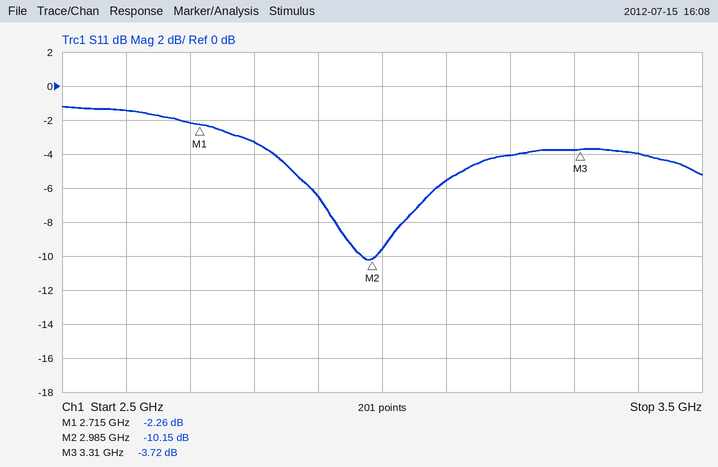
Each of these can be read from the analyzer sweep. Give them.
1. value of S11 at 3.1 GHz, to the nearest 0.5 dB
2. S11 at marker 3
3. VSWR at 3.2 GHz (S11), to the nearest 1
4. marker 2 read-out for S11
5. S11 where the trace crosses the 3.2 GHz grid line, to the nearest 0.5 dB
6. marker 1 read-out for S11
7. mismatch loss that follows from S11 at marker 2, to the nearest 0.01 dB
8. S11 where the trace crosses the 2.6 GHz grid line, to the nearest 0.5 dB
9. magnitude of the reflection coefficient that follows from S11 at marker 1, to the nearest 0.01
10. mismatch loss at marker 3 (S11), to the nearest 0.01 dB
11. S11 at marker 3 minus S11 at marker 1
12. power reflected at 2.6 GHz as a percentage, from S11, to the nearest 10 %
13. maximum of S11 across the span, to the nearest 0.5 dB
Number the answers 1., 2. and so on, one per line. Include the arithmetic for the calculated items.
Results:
1. -5.5 dB
2. -3.72 dB
3. |Γ| = 10^(-4/20) = 0.6310; VSWR = (1 + 0.6310)/(1 − 0.6310) ≈ 4
4. -10.15 dB
5. -4.0 dB
6. -2.26 dB
7. −10 log10(1 − 10^(-10.15/10)) ≈ 0.44 dB
8. -1.5 dB
9. 10^(-2.26/20) ≈ 0.77
10. −10 log10(1 − 10^(-3.72/10)) ≈ 2.40 dB
11. -3.72 − (-2.26) = -1.46 dB
12. 10^(-1.5/10) ≈ 70.8 %, so 70 % to the nearest 10 %
13. -1.0 dB
